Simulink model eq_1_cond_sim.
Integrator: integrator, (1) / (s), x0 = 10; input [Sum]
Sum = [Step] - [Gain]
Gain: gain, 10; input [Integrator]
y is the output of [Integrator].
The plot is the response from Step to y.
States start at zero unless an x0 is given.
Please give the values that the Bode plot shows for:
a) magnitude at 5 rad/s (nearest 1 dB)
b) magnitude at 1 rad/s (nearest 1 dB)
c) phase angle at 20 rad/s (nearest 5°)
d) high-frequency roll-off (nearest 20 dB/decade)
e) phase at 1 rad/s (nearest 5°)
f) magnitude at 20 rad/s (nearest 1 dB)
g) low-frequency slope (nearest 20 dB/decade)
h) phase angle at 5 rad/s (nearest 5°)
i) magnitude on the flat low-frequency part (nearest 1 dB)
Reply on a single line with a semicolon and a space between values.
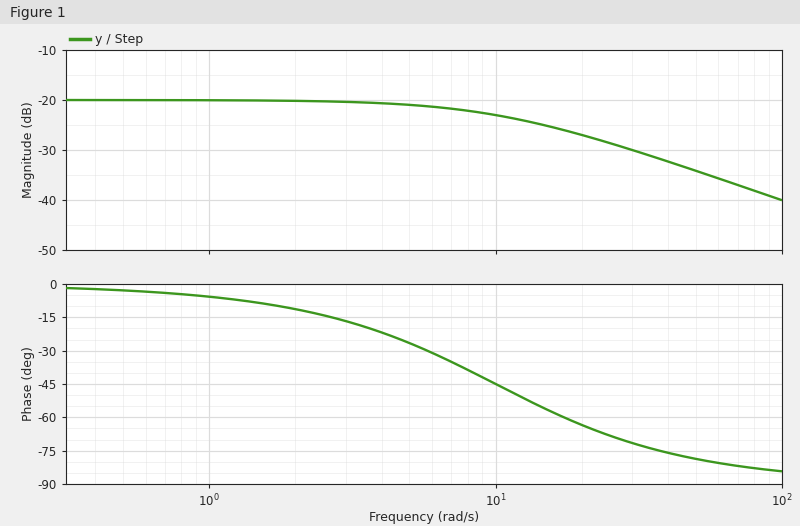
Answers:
-21 dB; -20 dB; -65°; -20 dB/decade; -5°; -27 dB; 0 dB/decade; -25°; -20 dB
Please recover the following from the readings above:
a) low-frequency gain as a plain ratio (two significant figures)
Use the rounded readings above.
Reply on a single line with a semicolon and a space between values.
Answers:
0.10
